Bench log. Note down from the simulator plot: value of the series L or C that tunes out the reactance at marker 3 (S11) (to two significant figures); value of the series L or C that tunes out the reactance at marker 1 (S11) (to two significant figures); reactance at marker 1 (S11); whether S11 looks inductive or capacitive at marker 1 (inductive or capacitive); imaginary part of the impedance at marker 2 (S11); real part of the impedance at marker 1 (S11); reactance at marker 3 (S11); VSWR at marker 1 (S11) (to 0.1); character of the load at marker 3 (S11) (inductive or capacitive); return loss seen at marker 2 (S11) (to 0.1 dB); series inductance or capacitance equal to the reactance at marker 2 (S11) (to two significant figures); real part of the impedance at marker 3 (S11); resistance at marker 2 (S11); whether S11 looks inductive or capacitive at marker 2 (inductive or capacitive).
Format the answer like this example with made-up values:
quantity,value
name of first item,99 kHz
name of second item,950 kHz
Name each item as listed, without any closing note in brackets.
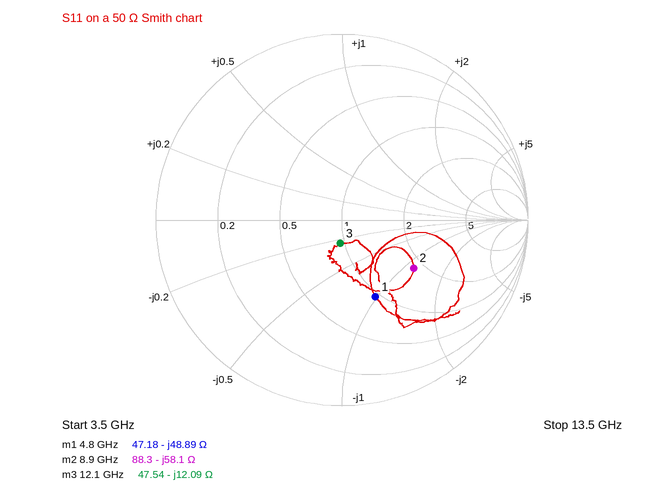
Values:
quantity,value
value of the series L or C that tunes out the reactance at marker 3 (S11),160 pH
value of the series L or C that tunes out the reactance at marker 1 (S11),1.6 nH
reactance at marker 1,-48.89 Ω
whether S11 looks inductive or capacitive at marker 1,capacitive
imaginary part of the impedance at marker 2,-58.1 Ω
real part of the impedance at marker 1,47.18 Ω
reactance at marker 3,-12.09 Ω
VSWR at marker 1 (S11),2.6
character of the load at marker 3 (S11),capacitive
return loss seen at marker 2 (S11),6.7 dB
series inductance or capacitance equal to the reactance at marker 2 (S11),310 fF
real part of the impedance at marker 3,47.54 Ω
resistance at marker 2,88.3 Ω
whether S11 looks inductive or capacitive at marker 2,capacitive
